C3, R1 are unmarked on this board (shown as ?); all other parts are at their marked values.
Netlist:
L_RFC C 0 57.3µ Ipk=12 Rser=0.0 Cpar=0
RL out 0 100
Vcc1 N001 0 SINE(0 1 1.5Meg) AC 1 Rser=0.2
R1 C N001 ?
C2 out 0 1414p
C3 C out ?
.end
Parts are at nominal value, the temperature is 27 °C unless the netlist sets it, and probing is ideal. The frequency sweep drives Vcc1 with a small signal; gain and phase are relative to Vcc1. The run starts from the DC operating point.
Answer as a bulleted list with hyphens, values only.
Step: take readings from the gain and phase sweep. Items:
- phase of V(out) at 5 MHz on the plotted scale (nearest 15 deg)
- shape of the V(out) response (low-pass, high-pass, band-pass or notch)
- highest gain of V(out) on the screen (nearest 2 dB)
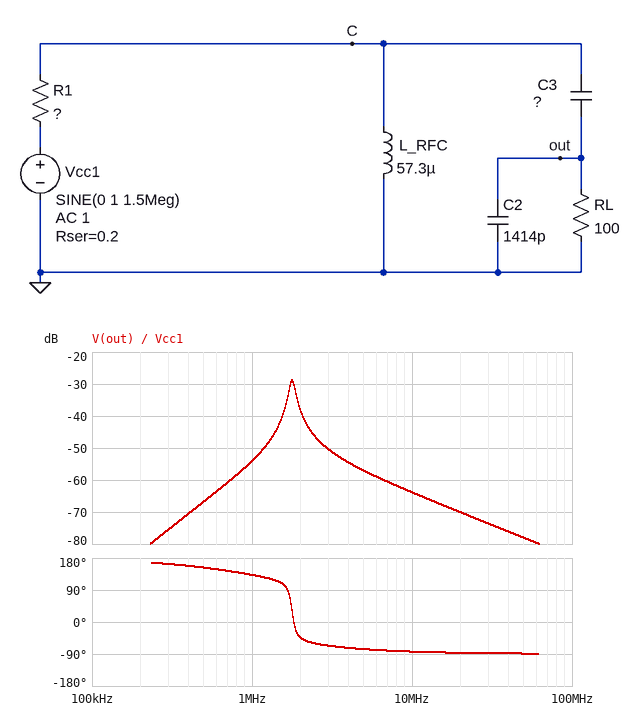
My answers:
- -75 deg
- band-pass
- -28 dB
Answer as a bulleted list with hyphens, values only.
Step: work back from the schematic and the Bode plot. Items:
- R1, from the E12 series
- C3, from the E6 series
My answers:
- 18 kΩ
- 150 pF
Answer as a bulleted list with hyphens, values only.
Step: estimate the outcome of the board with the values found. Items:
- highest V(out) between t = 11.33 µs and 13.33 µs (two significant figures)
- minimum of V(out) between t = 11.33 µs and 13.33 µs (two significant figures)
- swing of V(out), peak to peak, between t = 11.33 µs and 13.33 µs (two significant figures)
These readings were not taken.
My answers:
- 8.1 mV
- -8.1 mV
- 16 mV
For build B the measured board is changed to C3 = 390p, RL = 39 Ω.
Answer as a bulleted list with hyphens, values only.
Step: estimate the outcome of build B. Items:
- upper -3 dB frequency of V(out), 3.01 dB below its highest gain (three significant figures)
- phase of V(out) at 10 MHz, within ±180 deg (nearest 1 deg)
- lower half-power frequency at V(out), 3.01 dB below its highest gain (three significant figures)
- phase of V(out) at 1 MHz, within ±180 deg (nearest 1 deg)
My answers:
- 1.15 MHz
- -74 deg
- 1.03 MHz
- 125 deg
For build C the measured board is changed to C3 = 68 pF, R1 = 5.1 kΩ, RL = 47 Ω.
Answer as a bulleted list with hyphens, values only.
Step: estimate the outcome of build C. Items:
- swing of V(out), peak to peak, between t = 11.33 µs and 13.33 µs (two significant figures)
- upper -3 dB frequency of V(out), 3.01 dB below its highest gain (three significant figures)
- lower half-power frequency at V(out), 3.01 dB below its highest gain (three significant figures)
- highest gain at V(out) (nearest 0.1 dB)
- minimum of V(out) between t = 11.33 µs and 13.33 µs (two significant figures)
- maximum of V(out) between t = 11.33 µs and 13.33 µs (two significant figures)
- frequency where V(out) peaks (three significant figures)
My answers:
- 8.0 mV
- 2.89 MHz
- 2.35 MHz
- -30.3 dB
- -4.0 mV
- 4.0 mV
- 2.59 MHz
